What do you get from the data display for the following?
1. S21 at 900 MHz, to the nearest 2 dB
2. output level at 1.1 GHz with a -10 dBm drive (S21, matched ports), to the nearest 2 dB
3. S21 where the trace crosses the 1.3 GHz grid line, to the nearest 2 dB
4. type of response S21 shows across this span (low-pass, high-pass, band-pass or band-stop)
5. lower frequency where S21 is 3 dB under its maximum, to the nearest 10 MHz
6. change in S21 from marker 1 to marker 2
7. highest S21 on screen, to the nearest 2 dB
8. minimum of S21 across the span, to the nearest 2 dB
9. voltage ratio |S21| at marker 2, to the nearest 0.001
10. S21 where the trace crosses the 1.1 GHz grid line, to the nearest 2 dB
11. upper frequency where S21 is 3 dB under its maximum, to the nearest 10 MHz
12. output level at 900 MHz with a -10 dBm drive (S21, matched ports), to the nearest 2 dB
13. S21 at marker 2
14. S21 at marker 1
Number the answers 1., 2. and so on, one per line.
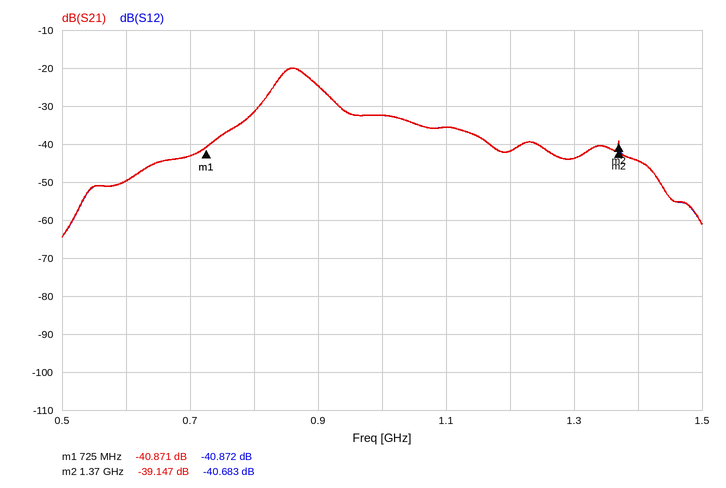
1. -24 dB
2. -46 dBm
3. -44 dB
4. band-pass
5. 840 MHz
6. 1.724 dB
7. -20 dB
8. -64 dB
9. 0.011
10. -36 dB
11. 890 MHz
12. -34 dBm
13. -39.147 dB
14. -40.871 dB
